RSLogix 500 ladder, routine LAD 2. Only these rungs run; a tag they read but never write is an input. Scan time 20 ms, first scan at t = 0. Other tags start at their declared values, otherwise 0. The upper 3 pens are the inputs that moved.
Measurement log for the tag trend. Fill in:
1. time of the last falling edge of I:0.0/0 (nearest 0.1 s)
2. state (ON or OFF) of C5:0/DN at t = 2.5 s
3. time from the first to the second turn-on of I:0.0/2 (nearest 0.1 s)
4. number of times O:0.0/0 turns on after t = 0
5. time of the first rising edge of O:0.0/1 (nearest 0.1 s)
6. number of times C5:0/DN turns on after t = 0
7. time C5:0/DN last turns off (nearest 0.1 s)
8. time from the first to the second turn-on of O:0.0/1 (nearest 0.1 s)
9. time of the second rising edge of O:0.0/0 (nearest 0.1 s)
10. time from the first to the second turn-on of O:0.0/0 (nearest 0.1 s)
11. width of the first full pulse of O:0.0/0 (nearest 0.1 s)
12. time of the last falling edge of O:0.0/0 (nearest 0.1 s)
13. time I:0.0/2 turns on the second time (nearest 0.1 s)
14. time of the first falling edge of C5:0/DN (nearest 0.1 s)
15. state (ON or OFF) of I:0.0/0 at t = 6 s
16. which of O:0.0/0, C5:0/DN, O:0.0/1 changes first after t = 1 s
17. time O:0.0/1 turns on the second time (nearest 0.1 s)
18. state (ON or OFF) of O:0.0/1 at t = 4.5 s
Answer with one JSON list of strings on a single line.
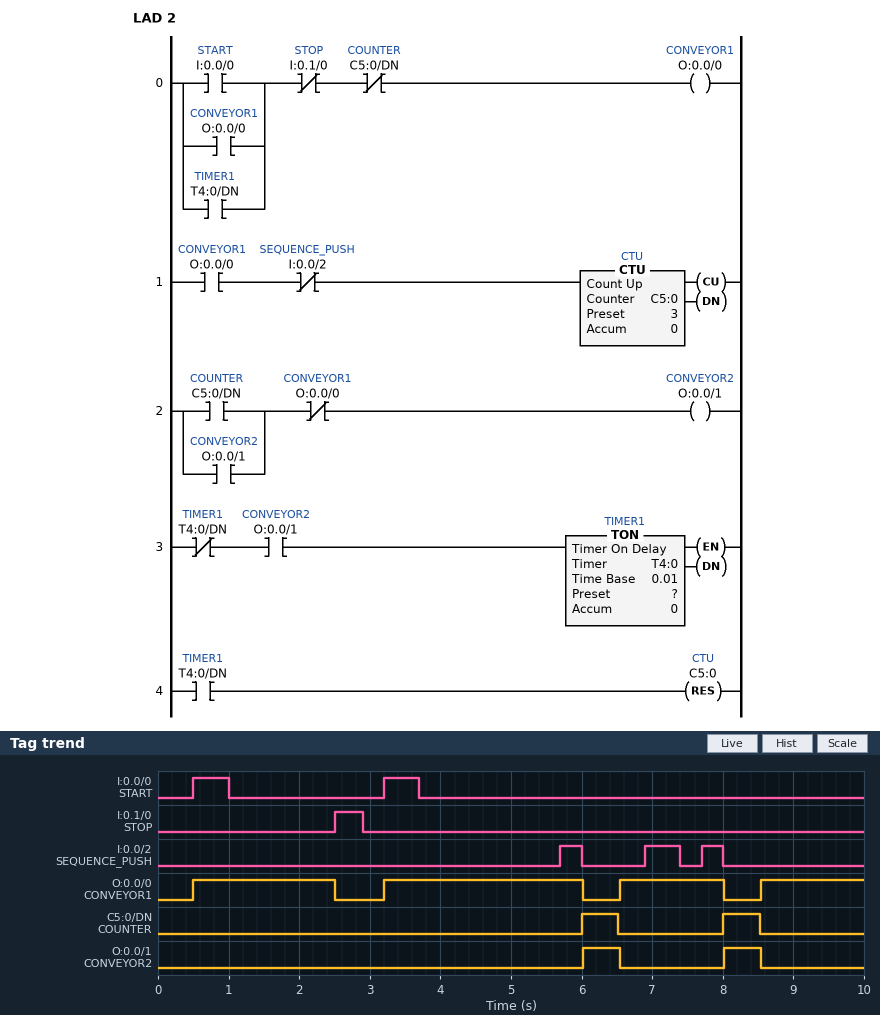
["3.7 s", "OFF", "1.2 s", "4", "6.0 s", "2", "8.5 s", "2.0 s", "3.2 s", "2.7 s", "2.0 s", "8.0 s", "6.9 s", "6.5 s", "OFF", "O:0.0/0", "8.0 s", "OFF"]
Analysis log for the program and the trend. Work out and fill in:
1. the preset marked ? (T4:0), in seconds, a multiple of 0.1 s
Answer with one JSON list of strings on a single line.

["0.5 s"]
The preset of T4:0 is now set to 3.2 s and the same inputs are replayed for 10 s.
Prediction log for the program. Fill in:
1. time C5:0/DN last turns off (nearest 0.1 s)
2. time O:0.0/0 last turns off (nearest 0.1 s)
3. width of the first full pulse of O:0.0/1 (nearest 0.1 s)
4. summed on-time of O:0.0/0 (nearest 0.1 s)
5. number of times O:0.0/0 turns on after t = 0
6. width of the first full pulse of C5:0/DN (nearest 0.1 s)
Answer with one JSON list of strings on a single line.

["9.2 s", "6.0 s", "3.2 s", "5.6 s", "3", "3.2 s"]
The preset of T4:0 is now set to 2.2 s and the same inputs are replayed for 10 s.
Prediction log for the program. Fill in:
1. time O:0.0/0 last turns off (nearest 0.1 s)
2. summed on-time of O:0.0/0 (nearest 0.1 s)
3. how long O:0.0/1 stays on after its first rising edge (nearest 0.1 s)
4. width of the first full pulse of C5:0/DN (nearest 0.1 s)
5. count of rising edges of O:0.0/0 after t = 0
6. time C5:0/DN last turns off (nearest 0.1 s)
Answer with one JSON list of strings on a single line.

["6.0 s", "6.6 s", "2.2 s", "2.2 s", "3", "8.2 s"]
